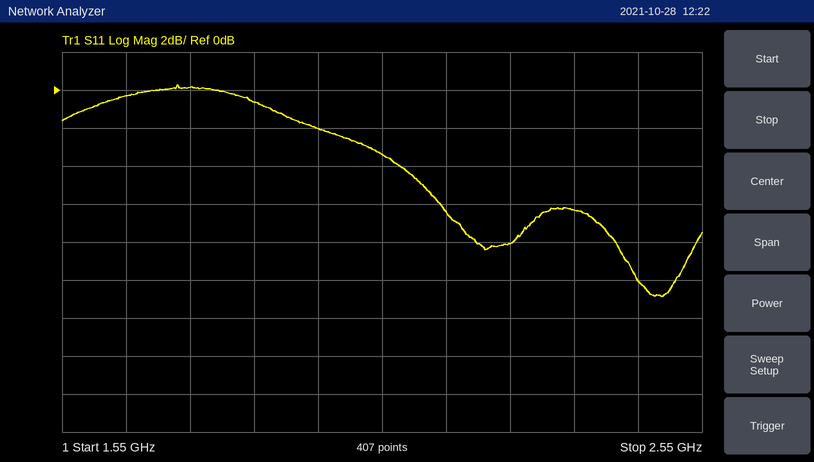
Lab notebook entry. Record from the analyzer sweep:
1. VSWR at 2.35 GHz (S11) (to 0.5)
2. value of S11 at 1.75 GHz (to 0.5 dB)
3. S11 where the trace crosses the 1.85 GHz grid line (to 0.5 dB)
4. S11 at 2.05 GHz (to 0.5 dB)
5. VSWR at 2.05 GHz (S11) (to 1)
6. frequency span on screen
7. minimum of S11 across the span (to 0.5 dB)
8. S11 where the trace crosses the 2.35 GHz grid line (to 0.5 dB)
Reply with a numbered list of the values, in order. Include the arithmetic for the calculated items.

1. |Γ| = 10^(-6.5/20) = 0.4732; VSWR = (1 + 0.4732)/(1 − 0.4732) ≈ 2.80, so 3.0 to the nearest 0.5
2. 0.0 dB
3. -0.5 dB
4. -3.5 dB
5. |Γ| = 10^(-3.5/20) = 0.6683; VSWR = (1 + 0.6683)/(1 − 0.6683) ≈ 5
6. 1 GHz
7. -11.0 dB
8. -6.5 dB
